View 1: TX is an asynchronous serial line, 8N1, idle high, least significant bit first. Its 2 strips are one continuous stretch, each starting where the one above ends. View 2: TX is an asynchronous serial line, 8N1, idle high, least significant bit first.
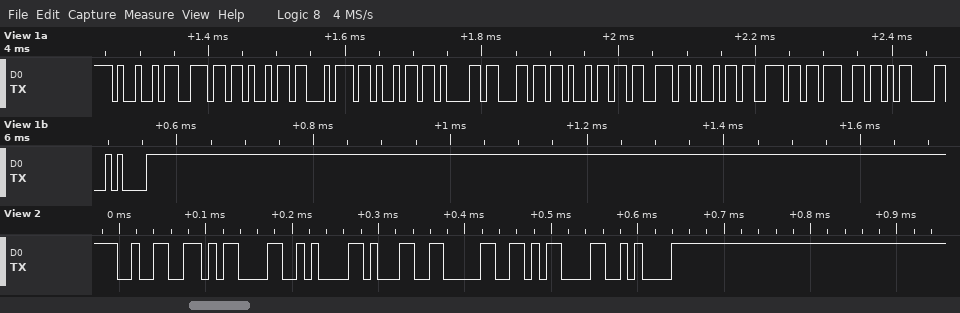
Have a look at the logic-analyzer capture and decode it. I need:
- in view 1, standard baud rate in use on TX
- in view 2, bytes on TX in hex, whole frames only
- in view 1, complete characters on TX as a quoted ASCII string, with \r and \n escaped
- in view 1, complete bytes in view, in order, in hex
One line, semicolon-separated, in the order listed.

115200 baud; 0x32 0x0D 0x0A 0x31 0x30 0x0D 0x0A; "Initialising\r\n"; 49 6E 69 74 69 61 6C 69 73 69 6E 67 0D 0A
